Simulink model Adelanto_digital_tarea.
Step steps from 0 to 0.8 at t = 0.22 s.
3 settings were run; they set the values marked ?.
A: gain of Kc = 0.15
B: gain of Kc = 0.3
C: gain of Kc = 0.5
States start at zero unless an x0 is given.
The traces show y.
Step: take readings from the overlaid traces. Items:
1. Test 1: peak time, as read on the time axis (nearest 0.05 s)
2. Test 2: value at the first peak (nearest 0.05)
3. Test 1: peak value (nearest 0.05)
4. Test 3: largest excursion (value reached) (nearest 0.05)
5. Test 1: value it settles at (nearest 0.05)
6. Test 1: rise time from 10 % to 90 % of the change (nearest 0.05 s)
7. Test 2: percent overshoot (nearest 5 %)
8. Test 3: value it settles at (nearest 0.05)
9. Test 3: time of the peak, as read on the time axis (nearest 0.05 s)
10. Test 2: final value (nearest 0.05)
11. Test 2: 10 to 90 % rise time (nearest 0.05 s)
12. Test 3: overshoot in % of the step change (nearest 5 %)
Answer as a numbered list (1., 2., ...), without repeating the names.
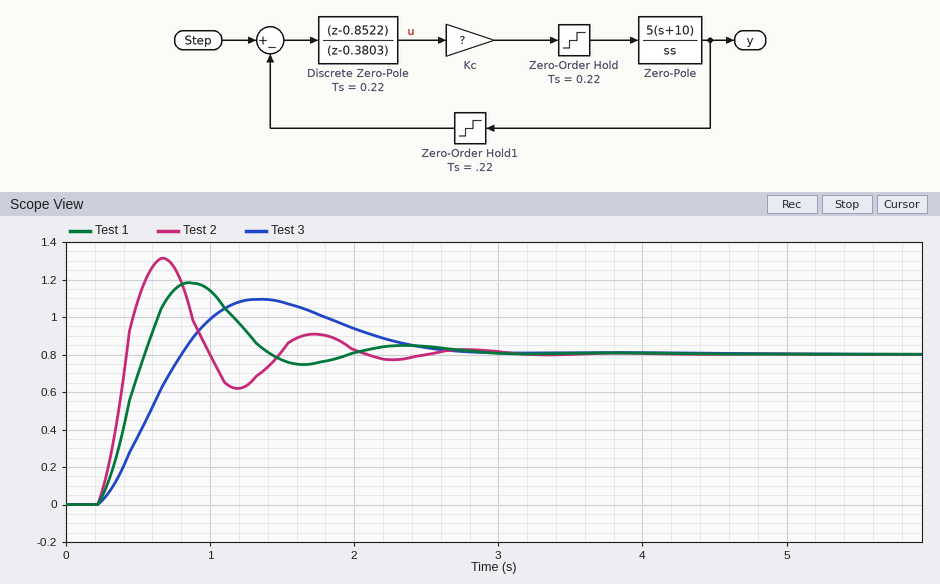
1. 0.85 s
2. 1.30
3. 1.20
4. 1.10
5. 0.80
6. 0.25 s
7. 65 %
8. 0.80
9. 1.35 s
10. 0.80
11. 0.15 s
12. 35 %
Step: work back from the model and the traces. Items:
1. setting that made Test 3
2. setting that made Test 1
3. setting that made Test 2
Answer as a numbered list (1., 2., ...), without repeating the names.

1. A
2. B
3. C
